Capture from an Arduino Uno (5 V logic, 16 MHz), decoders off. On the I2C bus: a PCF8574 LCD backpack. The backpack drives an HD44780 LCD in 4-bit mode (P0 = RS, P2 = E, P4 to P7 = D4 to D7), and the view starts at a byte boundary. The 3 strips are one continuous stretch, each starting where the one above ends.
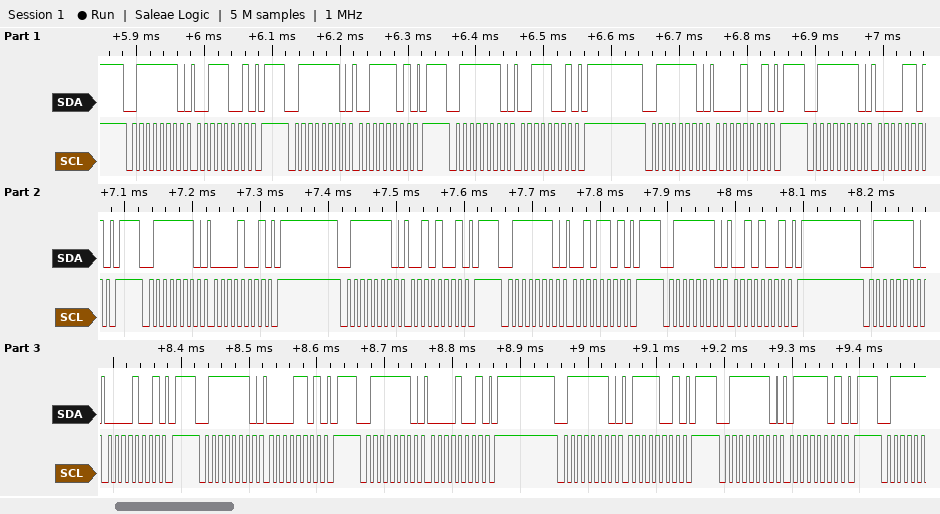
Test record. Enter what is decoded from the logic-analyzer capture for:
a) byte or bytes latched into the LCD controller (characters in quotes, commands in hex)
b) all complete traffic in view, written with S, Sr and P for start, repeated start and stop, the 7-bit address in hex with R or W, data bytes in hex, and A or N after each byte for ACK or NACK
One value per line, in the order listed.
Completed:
'0' ' '
S 3FW A 39 A P S 3FW A 3D A P S 3FW A 39 A P S 3FW A 09 A P S 3FW A 0D A P S 3FW A 09 A P S 3FW A 29 A P S 3FW A 2D A P S 3FW A 29 A P S 3FW A 09 A P S 3FW A 0D A P S 3FW A 09 A P S 3FW A 79 A P S 3FW A 7D A P
